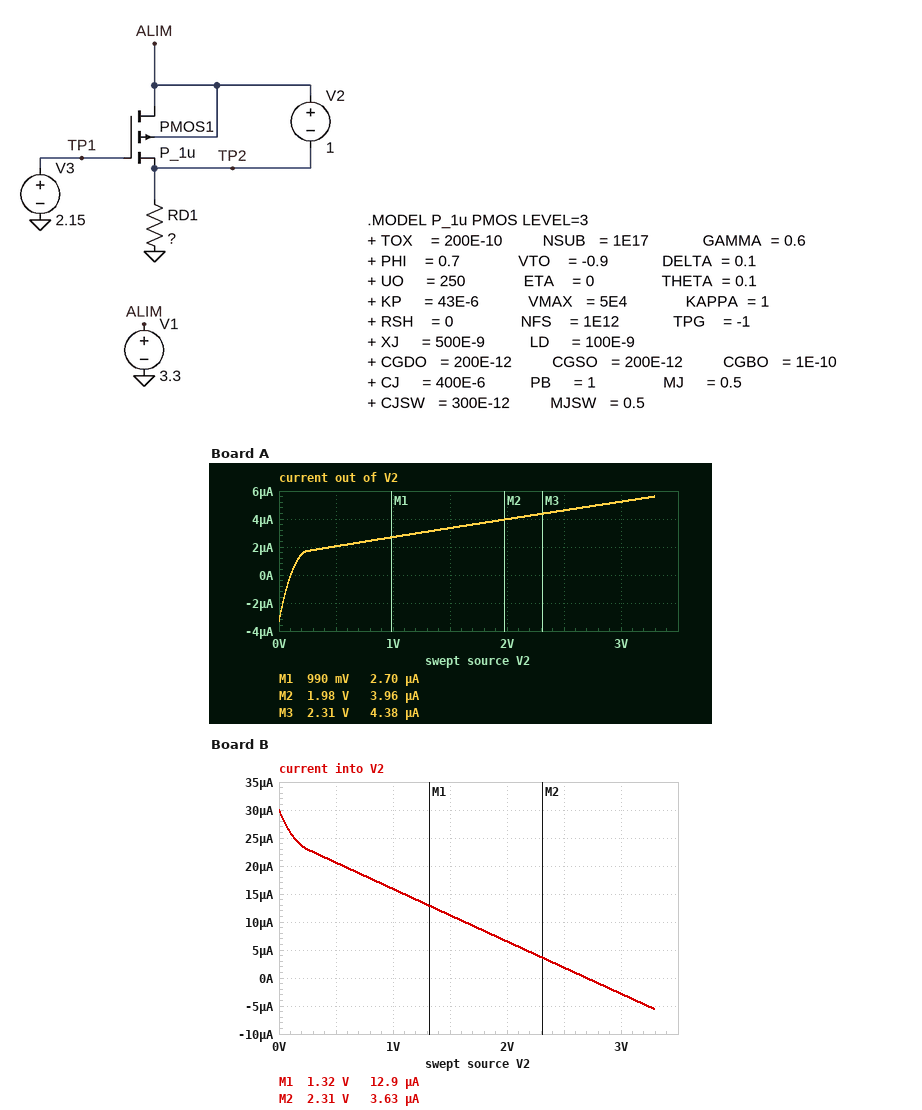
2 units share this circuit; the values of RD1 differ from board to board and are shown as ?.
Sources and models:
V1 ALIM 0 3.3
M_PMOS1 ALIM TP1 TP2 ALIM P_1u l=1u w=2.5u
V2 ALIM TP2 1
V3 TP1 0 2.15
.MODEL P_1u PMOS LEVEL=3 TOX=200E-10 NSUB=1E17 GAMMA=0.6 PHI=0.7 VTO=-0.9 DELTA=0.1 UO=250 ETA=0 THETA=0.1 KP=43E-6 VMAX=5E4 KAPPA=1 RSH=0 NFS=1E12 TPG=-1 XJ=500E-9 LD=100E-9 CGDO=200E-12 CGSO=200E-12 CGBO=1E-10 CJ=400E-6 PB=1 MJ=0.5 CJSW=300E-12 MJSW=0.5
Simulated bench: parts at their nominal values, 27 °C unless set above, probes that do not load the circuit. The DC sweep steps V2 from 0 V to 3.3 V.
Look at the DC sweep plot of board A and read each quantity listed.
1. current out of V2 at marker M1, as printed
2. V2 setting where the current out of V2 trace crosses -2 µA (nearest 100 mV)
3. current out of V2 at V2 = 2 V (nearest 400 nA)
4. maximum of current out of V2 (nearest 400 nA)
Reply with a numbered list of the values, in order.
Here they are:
1. 2.70 µA
2. 0 V
3. 4.0 µA
4. 5.6 µA
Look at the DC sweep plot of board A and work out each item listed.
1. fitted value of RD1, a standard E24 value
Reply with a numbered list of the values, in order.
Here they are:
1. 1 MΩ
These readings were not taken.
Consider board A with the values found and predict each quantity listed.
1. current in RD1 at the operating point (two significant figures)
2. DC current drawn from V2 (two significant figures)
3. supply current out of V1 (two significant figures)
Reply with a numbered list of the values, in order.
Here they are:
1. 2.3 µA
2. 2.7 µA
3. 2.3 µA
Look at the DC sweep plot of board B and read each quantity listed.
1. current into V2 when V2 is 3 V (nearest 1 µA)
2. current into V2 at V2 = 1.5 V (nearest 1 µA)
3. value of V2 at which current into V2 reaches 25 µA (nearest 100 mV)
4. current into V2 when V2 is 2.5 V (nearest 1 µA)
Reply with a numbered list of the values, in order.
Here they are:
1. -3 µA
2. 11 µA
3. 100 mV
4. 2 µA
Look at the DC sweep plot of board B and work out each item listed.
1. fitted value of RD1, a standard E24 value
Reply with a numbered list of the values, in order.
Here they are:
1. 110 kΩ
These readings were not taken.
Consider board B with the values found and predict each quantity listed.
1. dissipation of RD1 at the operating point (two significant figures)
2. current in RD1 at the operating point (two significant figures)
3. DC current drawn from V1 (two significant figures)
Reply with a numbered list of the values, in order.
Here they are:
1. 48 µW
2. 21 µA
3. 21 µA
